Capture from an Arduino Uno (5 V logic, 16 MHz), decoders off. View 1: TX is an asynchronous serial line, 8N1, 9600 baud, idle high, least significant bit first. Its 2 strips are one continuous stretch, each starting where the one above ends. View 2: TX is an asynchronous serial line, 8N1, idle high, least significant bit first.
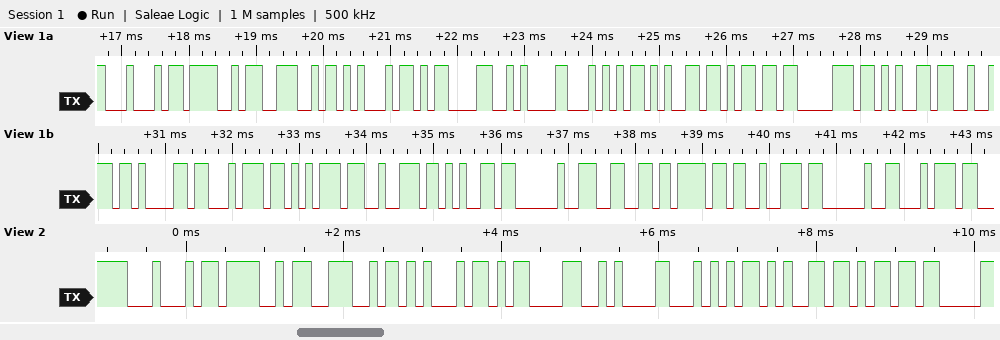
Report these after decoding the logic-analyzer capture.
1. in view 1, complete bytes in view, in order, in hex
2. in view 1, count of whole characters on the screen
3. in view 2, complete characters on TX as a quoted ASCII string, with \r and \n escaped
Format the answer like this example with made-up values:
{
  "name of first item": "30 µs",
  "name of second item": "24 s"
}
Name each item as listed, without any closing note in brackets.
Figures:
{
  "in view 1, complete bytes in view, in order, in hex": "0x44 0x4F 0x4E 0x45 0x0D 0x0A 0x54 0x65 0x6D 0x70 0x65 0x72 0x61 0x74 0x75 0x72 0x65 0x20 0x66 0x6F 0x72 0x20 0x74",
  "in view 1, count of whole characters on the screen": "23",
  "in view 2, complete characters on TX as a quoted ASCII string, with \\r and \\n escaped": "\"DONE\\r\\nTem\""
}
